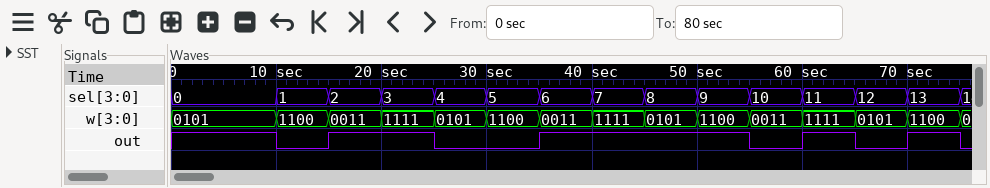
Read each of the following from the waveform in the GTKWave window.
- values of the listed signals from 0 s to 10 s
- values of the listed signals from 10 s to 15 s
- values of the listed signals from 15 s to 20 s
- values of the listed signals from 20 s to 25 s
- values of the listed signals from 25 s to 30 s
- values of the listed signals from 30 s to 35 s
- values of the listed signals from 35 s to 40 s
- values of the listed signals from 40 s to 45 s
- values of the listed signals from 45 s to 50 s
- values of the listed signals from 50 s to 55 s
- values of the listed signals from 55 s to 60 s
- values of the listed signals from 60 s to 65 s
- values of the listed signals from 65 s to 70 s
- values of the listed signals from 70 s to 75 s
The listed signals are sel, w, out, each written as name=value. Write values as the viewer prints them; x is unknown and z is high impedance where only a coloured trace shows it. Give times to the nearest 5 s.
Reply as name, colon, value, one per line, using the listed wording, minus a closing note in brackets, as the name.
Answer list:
values of the listed signals from 0 s to 10 s: sel=0, w=0101, out=1
values of the listed signals from 10 s to 15 s: sel=1, w=1100, out=0
values of the listed signals from 15 s to 20 s: sel=2, w=0011, out=1
values of the listed signals from 20 s to 25 s: sel=3, w=1111, out=1
values of the listed signals from 25 s to 30 s: sel=4, w=0101, out=0
values of the listed signals from 30 s to 35 s: sel=5, w=1100, out=0
values of the listed signals from 35 s to 40 s: sel=6, w=0011, out=1
values of the listed signals from 40 s to 45 s: sel=7, w=1111, out=1
values of the listed signals from 45 s to 50 s: sel=8, w=0101, out=1
values of the listed signals from 50 s to 55 s: sel=9, w=1100, out=1
values of the listed signals from 55 s to 60 s: sel=10, w=0011, out=0
values of the listed signals from 60 s to 65 s: sel=11, w=1111, out=1
values of the listed signals from 65 s to 70 s: sel=12, w=0101, out=0
values of the listed signals from 70 s to 75 s: sel=13, w=1100, out=1
